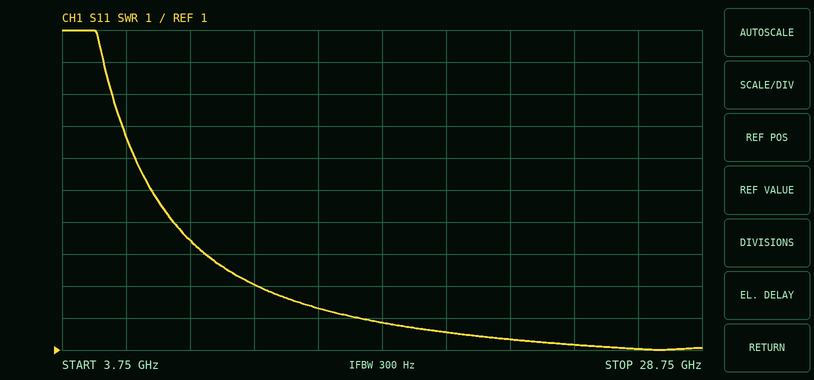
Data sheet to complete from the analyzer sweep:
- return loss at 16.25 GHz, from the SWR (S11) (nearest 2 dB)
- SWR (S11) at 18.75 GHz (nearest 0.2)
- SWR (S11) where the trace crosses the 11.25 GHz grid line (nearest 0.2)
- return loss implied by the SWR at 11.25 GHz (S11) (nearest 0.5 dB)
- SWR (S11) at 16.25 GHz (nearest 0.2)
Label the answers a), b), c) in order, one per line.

a) 10 dB
b) 1.6
c) 3.0
d) 6.0 dB
e) 1.8
